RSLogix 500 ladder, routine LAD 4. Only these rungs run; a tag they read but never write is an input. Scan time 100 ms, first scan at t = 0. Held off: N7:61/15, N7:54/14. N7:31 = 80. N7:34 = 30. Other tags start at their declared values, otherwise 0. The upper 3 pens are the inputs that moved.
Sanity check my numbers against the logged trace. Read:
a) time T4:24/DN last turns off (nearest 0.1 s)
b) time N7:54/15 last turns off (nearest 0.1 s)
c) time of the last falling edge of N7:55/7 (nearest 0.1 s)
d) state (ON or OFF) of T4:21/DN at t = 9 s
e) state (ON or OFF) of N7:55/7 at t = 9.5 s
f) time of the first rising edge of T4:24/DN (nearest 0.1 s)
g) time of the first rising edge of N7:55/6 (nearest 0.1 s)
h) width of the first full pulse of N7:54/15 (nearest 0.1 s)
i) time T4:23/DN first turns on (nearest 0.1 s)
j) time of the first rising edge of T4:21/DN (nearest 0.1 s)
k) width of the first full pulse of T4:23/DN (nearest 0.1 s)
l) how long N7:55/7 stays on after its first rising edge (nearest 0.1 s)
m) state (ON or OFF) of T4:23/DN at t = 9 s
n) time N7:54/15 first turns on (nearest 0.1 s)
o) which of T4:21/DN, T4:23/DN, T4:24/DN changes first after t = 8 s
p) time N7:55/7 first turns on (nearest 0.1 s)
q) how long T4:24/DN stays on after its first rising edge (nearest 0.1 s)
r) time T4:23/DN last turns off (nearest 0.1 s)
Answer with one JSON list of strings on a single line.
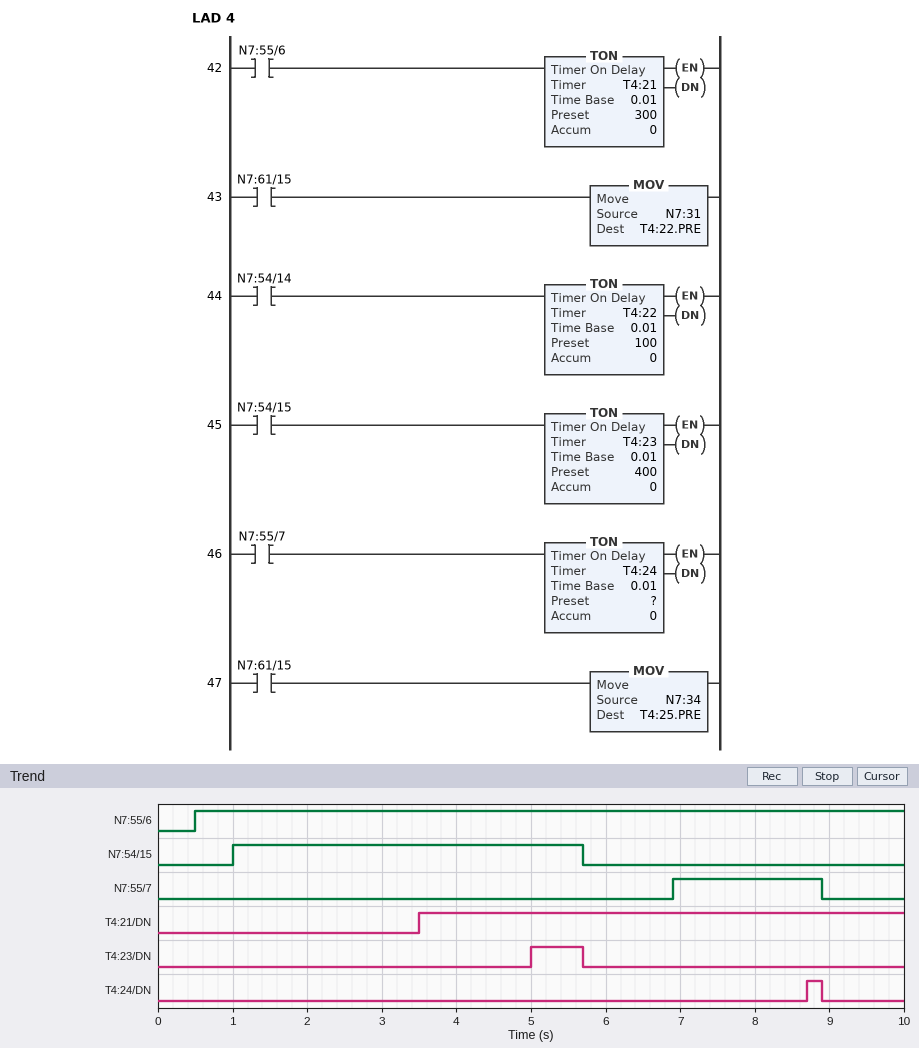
["8.9 s", "5.7 s", "8.9 s", "ON", "OFF", "8.7 s", "0.5 s", "4.7 s", "5.0 s", "3.5 s", "0.7 s", "2.0 s", "OFF", "1.0 s", "T4:24/DN", "6.9 s", "0.2 s", "5.7 s"]
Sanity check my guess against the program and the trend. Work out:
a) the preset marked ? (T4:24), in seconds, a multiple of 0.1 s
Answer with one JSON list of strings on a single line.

["1.8 s"]
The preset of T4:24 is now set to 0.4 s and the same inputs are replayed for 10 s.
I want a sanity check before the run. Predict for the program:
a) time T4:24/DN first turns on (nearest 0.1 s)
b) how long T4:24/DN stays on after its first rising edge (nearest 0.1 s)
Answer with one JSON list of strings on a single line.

["7.3 s", "1.6 s"]
